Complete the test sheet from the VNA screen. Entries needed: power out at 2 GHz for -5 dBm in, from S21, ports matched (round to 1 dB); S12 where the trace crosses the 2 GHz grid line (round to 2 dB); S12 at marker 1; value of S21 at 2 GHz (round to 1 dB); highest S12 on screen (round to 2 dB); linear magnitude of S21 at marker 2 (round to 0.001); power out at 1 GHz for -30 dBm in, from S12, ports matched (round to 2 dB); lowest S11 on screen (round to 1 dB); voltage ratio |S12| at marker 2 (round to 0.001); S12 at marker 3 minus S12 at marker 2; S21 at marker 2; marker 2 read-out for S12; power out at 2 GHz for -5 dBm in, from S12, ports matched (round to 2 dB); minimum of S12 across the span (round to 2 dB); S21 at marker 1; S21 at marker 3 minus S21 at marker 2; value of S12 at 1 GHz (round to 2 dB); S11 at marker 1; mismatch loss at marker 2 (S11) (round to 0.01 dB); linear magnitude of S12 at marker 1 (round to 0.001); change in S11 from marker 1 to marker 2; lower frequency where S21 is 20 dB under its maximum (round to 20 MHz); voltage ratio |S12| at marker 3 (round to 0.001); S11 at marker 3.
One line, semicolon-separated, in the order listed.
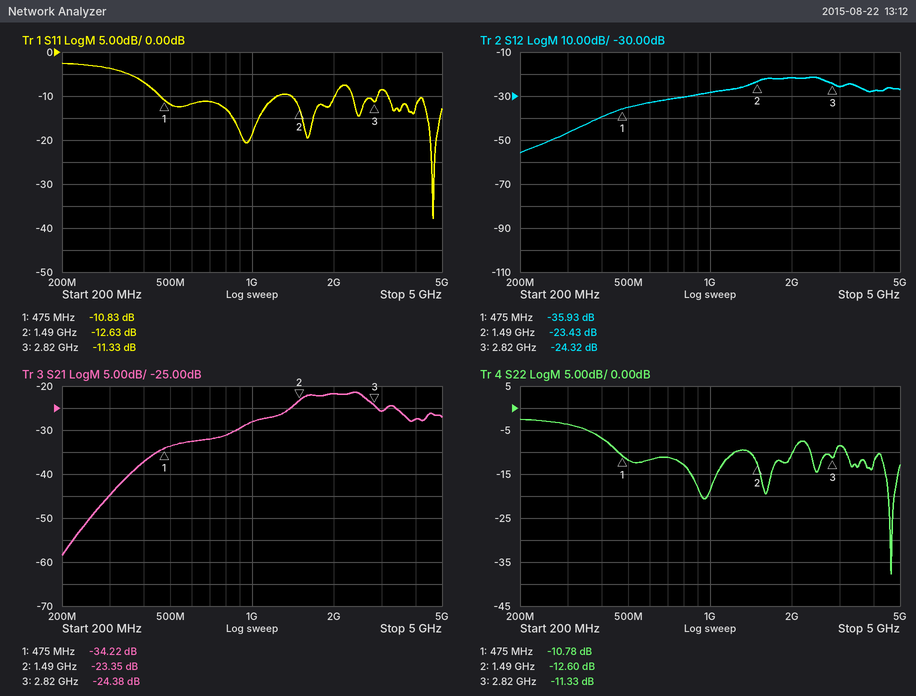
-27 dBm; -22 dB; -35.93 dB; -22 dB; -22 dB; 0.068; -58 dBm; -38 dB; 0.067; -0.89 dB; -23.35 dB; -23.43 dB; -26 dBm; -56 dB; -34.22 dB; -1.03 dB; -28 dB; -10.83 dB; 0.24 dB; 0.016; -1.80 dB; 340 MHz; 0.061; -11.33 dB
